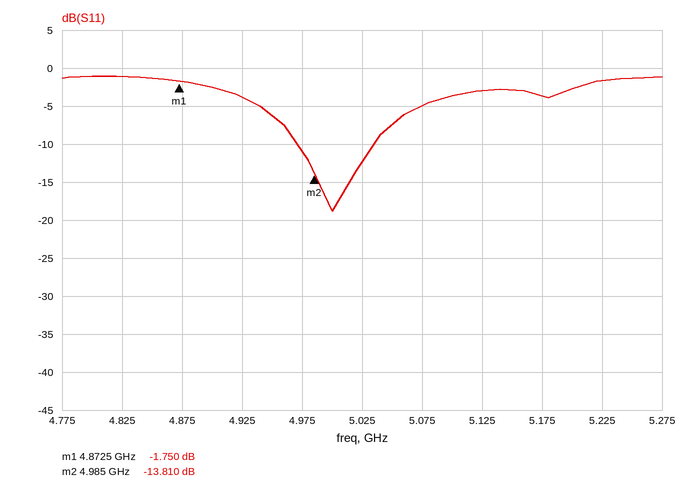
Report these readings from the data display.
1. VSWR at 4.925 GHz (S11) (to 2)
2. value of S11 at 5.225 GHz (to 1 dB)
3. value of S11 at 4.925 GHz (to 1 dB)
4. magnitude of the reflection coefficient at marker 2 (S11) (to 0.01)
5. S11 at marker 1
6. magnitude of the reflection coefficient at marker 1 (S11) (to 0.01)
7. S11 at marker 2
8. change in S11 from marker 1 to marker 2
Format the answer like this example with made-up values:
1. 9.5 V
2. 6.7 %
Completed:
1. 4
2. -2 dB
3. -4 dB
4. 0.20
5. -1.750 dB
6. 0.82
7. -13.810 dB
8. -12.060 dB
